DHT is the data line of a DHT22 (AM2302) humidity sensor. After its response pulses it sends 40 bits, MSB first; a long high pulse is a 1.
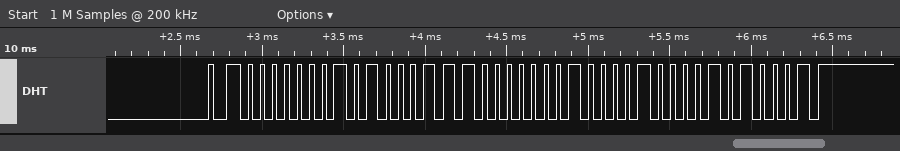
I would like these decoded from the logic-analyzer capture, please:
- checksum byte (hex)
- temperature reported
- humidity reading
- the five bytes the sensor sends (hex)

0x51
26.4 °C
32.7 %
01 47 01 08 51
